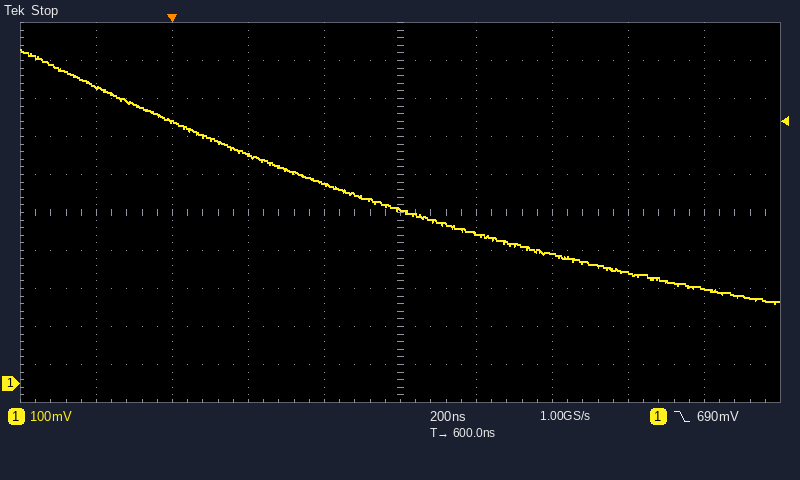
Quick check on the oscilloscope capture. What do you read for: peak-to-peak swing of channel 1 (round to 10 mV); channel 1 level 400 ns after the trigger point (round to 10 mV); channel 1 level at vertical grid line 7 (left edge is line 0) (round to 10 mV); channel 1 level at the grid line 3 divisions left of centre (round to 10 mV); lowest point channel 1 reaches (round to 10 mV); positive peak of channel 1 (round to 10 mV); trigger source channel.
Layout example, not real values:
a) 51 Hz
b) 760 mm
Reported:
a) 670 mV
b) 530 mV
c) 340 mV
d) 690 mV
e) 210 mV
f) 880 mV
g) channel 1
